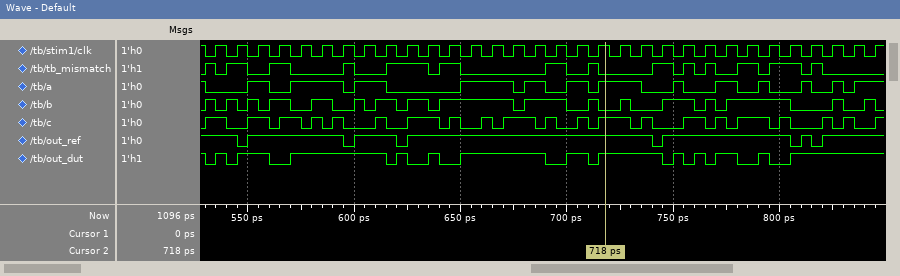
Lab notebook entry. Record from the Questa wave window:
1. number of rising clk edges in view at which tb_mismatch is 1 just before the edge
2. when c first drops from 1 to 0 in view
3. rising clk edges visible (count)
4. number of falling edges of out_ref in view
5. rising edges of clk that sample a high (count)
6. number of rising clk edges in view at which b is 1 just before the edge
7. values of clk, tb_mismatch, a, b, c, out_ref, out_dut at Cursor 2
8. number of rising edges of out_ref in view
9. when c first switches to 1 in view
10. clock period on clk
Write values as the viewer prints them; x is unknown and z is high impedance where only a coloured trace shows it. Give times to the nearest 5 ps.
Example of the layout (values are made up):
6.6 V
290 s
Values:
11
540 ps
32
6
18
20
clk=1, tb_mismatch=0, a=1, b=0, c=1, out_ref=1, out_dut=1
6
530 ps
10 ps
